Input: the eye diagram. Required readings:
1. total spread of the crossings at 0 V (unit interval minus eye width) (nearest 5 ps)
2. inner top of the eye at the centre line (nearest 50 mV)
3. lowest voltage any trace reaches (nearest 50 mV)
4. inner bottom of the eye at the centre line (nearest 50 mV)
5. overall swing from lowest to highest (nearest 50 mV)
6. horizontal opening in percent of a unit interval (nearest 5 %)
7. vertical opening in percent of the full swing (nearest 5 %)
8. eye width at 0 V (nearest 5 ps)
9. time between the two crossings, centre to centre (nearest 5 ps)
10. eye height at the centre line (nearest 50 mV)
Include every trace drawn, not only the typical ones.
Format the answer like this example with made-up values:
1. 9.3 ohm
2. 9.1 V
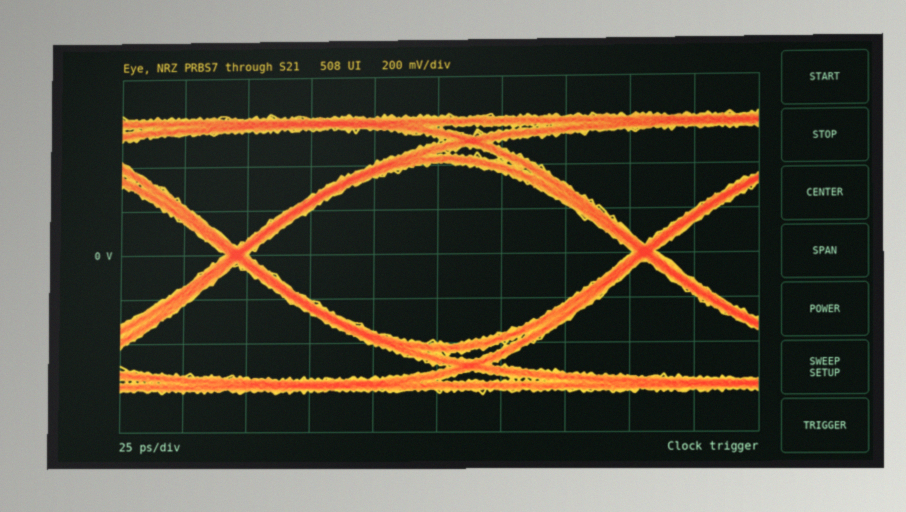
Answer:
1. 10 ps
2. 400 mV
3. -650 mV
4. -400 mV
5. 1.25 V
6. 95 %
7. 65 %
8. 150 ps
9. 160 ps
10. 800 mV
